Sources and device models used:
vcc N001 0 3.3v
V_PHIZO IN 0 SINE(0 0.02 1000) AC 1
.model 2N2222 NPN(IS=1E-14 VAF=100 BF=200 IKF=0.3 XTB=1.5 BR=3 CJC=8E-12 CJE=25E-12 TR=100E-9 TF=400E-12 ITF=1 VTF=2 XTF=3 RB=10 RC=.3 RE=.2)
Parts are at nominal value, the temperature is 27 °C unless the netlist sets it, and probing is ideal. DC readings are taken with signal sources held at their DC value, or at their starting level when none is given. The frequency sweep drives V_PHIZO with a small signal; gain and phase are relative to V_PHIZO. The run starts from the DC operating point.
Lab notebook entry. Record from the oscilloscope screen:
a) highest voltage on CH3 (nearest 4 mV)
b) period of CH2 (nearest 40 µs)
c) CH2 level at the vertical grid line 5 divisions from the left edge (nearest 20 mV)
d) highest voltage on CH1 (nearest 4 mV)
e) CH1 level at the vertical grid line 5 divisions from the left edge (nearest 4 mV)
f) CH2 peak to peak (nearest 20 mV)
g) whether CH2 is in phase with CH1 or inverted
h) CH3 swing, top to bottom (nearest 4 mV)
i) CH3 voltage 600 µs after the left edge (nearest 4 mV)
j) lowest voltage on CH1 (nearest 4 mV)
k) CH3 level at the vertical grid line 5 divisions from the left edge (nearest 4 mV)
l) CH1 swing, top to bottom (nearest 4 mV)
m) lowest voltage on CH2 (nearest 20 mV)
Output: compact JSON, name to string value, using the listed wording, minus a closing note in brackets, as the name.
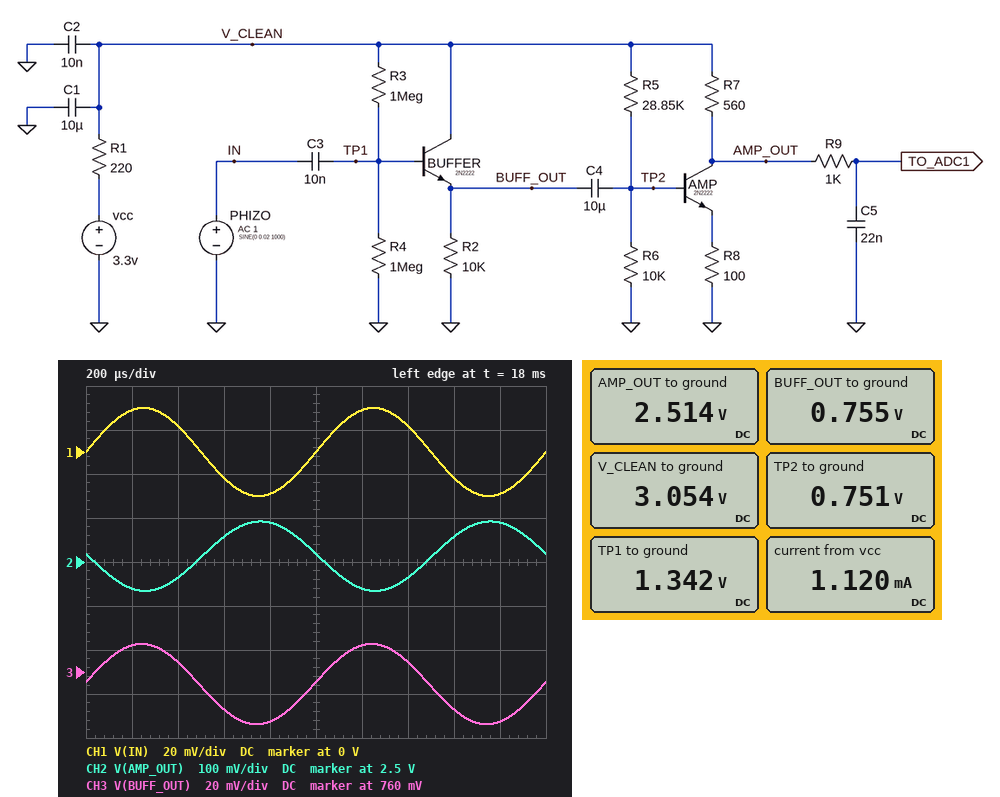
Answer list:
{"highest voltage on CH3": "772 mV", "period of CH2": "1.00 ms", "CH2 level at the vertical grid line 5 divisions from the left edge": "2.52 V", "highest voltage on CH1": "20 mV", "CH1 level at the vertical grid line 5 divisions from the left edge": "0 V", "CH2 peak to peak": "160 mV", "whether CH2 is in phase with CH1 or inverted": "inverted", "CH3 swing, top to bottom": "36 mV", "CH3 voltage 600 µs after the left edge": "744 mV", "lowest voltage on CH1": "-20 mV", "CH3 level at the vertical grid line 5 divisions from the left edge": "756 mV", "CH1 swing, top to bottom": "40 mV", "lowest voltage on CH2": "2.44 V"}
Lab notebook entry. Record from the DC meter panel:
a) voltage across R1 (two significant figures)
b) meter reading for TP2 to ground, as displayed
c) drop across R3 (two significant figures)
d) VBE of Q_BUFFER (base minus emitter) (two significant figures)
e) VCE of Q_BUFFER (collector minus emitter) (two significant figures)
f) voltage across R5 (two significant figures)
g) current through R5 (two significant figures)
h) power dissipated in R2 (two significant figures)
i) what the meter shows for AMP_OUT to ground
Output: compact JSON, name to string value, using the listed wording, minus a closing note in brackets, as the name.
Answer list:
{"voltage across R1": "250 mV", "meter reading for TP2 to ground, as displayed": "0.751 V", "drop across R3": "1.7 V", "VBE of Q_BUFFER (base minus emitter)": "590 mV", "VCE of Q_BUFFER (collector minus emitter)": "2.3 V", "voltage across R5": "2.3 V", "current through R5": "80 µA", "power dissipated in R2": "57 µW", "what the meter shows for AMP_OUT to ground": "2.514 V"}
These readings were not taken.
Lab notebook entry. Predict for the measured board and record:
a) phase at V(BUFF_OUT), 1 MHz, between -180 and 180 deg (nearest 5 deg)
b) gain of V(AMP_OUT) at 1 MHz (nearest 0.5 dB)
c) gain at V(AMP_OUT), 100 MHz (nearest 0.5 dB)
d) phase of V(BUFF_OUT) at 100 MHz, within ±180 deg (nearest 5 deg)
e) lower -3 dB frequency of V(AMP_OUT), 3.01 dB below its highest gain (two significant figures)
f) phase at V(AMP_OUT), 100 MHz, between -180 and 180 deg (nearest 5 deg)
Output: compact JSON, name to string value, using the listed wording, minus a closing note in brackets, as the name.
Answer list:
{"phase at V(BUFF_OUT), 1 MHz, between -180 and 180 deg": "-5 deg", "gain of V(AMP_OUT) at 1 MHz": "8.0 dB", "gain at V(AMP_OUT), 100 MHz": "2.5 dB", "phase of V(BUFF_OUT) at 100 MHz, within ±180 deg": "10 deg", "lower -3 dB frequency of V(AMP_OUT), 3.01 dB below its highest gain": "49 Hz", "phase at V(AMP_OUT), 100 MHz, between -180 and 180 deg": "85 deg"}
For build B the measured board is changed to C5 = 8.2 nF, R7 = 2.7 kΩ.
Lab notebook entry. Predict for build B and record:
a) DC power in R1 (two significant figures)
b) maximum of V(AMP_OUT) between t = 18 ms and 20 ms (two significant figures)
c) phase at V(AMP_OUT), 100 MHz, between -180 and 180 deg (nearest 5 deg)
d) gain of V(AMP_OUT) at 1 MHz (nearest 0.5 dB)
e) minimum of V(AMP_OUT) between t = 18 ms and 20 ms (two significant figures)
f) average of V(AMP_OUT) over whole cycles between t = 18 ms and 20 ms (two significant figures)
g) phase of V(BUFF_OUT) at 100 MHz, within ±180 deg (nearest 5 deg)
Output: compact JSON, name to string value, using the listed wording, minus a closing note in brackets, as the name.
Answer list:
{"DC power in R1": "270 µW", "maximum of V(AMP_OUT) between t = 18 ms and 20 ms": "880 mV", "phase at V(AMP_OUT), 100 MHz, between -180 and 180 deg": "55 deg", "gain of V(AMP_OUT) at 1 MHz": "14.0 dB", "minimum of V(AMP_OUT) between t = 18 ms and 20 ms": "210 mV", "average of V(AMP_OUT) over whole cycles between t = 18 ms and 20 ms": "520 mV", "phase of V(BUFF_OUT) at 100 MHz, within ±180 deg": "15 deg"}
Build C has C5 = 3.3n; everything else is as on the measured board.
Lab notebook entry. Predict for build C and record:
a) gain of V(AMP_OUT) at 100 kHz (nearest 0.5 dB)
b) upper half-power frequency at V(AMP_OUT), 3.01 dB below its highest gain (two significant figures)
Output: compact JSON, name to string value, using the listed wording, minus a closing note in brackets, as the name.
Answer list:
{"gain of V(AMP_OUT) at 100 kHz": "8.5 dB", "upper half-power frequency at V(AMP_OUT), 3.01 dB below its highest gain": "45 kHz"}
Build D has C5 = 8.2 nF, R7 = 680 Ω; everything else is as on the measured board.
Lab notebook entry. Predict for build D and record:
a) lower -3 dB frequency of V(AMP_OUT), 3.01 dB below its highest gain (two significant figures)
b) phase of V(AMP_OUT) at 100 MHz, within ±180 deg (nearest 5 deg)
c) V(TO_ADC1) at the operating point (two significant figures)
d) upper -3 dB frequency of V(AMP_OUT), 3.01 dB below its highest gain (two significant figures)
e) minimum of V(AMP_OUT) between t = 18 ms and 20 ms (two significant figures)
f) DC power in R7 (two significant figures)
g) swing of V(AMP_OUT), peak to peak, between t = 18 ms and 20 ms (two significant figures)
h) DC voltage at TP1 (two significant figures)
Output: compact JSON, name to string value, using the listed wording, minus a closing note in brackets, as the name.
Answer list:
{"lower -3 dB frequency of V(AMP_OUT), 3.01 dB below its highest gain": "51 Hz", "phase of V(AMP_OUT) at 100 MHz, within ±180 deg": "80 deg", "V(TO_ADC1) at the operating point": "2.4 V", "upper -3 dB frequency of V(AMP_OUT), 3.01 dB below its highest gain": "16 kHz", "minimum of V(AMP_OUT) between t = 18 ms and 20 ms": "2.3 V", "DC power in R7": "630 µW", "swing of V(AMP_OUT), peak to peak, between t = 18 ms and 20 ms": "190 mV", "DC voltage at TP1": "1.3 V"}
